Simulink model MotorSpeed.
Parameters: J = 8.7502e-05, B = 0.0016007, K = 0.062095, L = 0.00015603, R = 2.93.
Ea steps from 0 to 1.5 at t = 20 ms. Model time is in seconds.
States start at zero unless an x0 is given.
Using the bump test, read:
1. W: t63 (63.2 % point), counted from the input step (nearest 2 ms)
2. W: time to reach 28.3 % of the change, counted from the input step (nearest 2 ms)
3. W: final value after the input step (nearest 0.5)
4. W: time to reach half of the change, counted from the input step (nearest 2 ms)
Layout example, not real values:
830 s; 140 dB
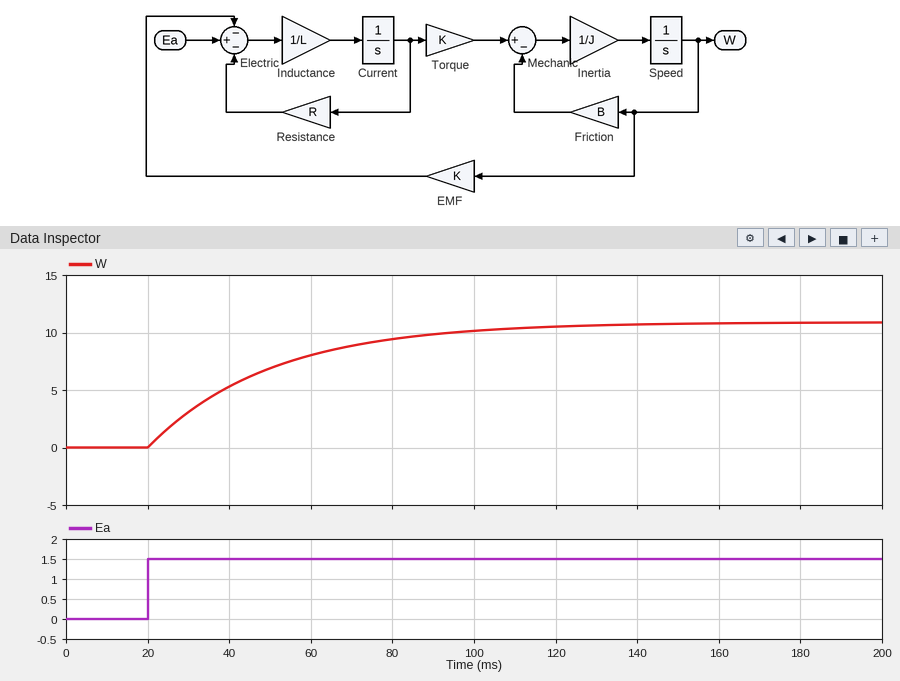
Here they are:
30 ms; 10 ms; 11.0; 20 ms
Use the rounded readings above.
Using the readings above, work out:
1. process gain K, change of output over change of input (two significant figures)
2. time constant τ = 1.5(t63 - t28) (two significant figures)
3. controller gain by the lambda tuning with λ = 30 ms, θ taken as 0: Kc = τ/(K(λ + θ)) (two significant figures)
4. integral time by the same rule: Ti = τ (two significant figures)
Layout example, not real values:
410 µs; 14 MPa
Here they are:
7.3; 30 ms; 0.14; 30 ms
